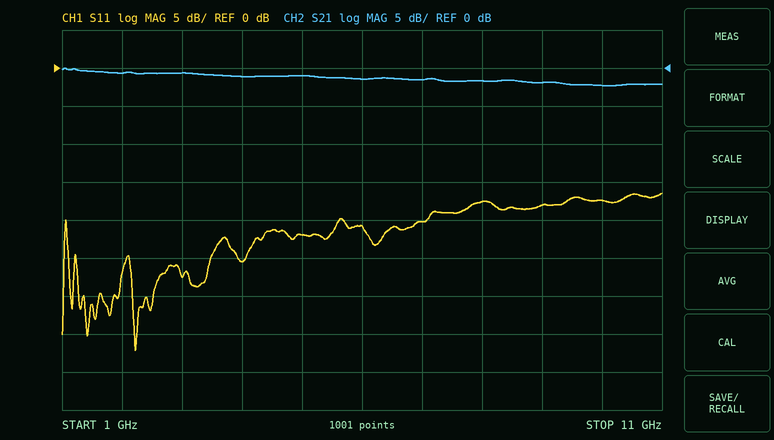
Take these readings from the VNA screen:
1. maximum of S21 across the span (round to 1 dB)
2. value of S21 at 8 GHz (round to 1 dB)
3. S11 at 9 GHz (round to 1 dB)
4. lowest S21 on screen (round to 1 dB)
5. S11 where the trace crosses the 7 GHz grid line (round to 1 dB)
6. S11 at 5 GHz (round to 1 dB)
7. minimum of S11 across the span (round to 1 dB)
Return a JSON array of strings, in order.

["0 dB", "-2 dB", "-18 dB", "-2 dB", "-20 dB", "-22 dB", "-37 dB"]
